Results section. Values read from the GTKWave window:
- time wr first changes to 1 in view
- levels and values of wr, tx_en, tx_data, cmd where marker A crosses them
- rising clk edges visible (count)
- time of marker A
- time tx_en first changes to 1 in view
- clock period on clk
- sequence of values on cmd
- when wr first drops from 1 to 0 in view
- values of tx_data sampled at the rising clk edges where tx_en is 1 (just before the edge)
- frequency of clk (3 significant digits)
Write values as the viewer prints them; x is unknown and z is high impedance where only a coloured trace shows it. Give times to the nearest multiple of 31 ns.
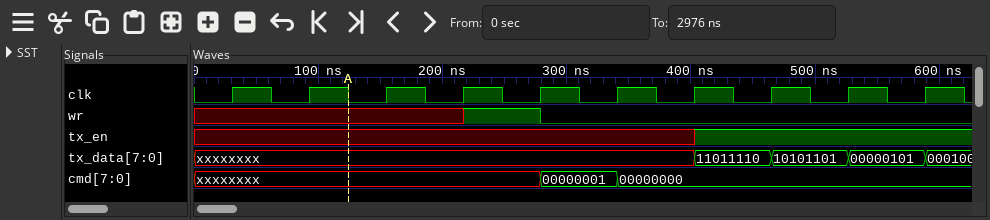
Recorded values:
217 ns
wr=x, tx_en=x, tx_data=xxxxxxxx, cmd=xxxxxxxx
10
124 ns
403 ns
62 ns
xxxxxxxx, 00000001, 00000000
279 ns
11011110, 10101101, 00000101
16.1 MHz
